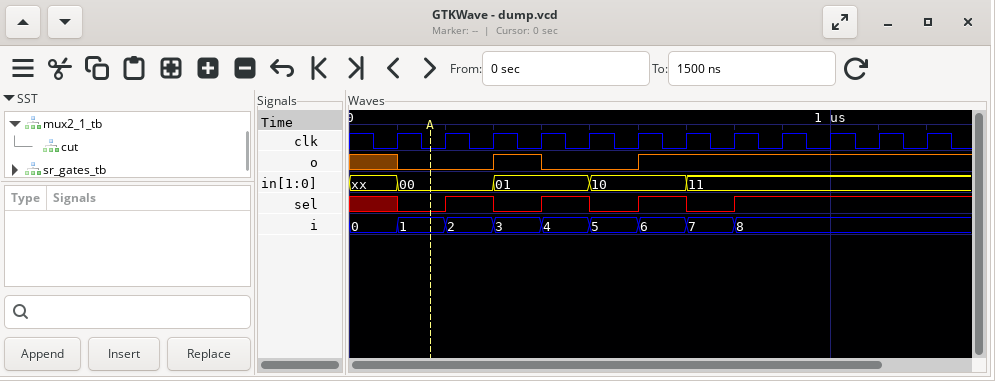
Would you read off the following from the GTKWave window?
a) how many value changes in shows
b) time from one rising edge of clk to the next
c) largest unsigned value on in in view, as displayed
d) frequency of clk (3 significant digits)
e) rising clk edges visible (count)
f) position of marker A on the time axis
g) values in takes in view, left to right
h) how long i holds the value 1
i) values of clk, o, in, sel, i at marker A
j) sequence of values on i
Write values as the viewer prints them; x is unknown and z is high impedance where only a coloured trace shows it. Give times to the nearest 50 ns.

4
100 ns
11
10.0 MHz
12
150 ns
xx, 00, 01, 10, 11
100 ns
clk=0, o=0, in=00, sel=0, i=1
0, 1, 2, 3, 4, 5, 6, 7, 8
